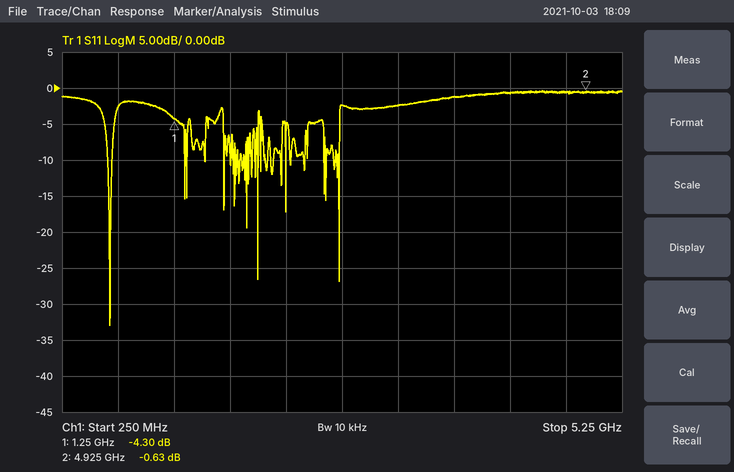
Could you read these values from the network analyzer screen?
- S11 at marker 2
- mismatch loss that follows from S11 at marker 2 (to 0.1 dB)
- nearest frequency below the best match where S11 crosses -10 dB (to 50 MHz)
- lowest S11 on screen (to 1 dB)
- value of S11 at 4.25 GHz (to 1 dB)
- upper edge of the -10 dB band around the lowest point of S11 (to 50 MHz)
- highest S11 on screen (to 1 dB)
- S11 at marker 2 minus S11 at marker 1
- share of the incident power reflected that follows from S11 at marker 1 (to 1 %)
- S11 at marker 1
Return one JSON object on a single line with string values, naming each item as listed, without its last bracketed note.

{"S11 at marker 2": "-0.63 dB", "mismatch loss that follows from S11 at marker 2": "8.7 dB", "nearest frequency below the best match where S11 crosses -10 dB": "650 MHz", "lowest S11 on screen": "-33 dB", "value of S11 at 4.25 GHz": "-1 dB", "upper edge of the -10 dB band around the lowest point of S11": "700 MHz", "highest S11 on screen": "0 dB", "S11 at marker 2 minus S11 at marker 1": "3.67 dB", "share of the incident power reflected that follows from S11 at marker 1": "37 %", "S11 at marker 1": "-4.30 dB"}
